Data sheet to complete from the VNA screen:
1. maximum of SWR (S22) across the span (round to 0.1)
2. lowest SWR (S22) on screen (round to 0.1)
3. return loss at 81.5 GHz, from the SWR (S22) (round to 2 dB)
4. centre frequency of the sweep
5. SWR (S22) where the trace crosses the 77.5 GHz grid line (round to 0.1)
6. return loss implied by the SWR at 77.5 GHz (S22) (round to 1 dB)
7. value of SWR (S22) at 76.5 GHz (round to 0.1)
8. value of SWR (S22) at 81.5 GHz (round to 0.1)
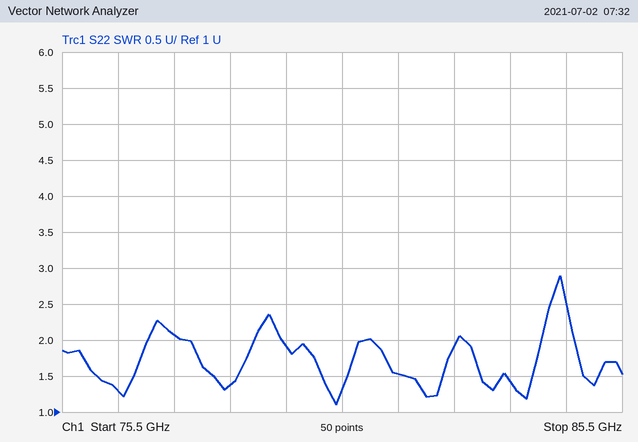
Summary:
2.9
1.1
14 dB
80.5 GHz
2.1
9 dB
1.3
1.5
